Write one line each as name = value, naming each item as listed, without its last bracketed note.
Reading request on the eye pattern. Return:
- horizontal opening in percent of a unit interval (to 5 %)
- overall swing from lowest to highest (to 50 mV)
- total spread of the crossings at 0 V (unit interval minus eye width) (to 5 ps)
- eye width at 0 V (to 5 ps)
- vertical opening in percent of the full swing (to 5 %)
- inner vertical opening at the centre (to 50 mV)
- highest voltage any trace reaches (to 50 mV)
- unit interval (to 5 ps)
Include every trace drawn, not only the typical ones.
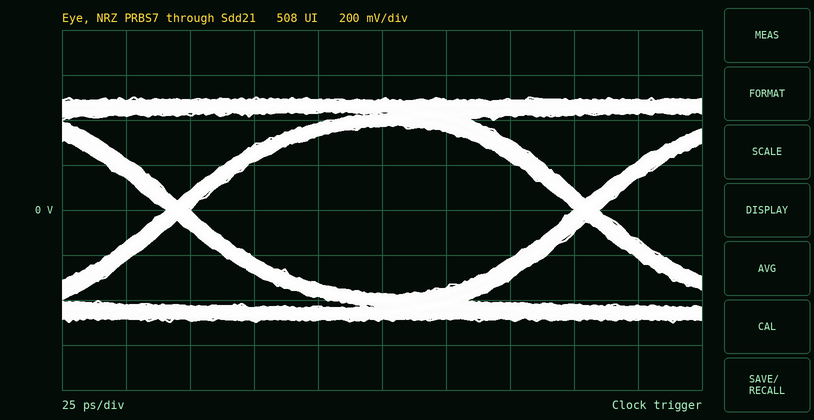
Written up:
horizontal opening in percent of a unit interval = 95 %
overall swing from lowest to highest = 1.00 V
total spread of the crossings at 0 V (unit interval minus eye width) = 10 ps
eye width at 0 V = 150 ps
vertical opening in percent of the full swing = 75 %
inner vertical opening at the centre = 750 mV
highest voltage any trace reaches = 500 mV
unit interval = 160 ps
